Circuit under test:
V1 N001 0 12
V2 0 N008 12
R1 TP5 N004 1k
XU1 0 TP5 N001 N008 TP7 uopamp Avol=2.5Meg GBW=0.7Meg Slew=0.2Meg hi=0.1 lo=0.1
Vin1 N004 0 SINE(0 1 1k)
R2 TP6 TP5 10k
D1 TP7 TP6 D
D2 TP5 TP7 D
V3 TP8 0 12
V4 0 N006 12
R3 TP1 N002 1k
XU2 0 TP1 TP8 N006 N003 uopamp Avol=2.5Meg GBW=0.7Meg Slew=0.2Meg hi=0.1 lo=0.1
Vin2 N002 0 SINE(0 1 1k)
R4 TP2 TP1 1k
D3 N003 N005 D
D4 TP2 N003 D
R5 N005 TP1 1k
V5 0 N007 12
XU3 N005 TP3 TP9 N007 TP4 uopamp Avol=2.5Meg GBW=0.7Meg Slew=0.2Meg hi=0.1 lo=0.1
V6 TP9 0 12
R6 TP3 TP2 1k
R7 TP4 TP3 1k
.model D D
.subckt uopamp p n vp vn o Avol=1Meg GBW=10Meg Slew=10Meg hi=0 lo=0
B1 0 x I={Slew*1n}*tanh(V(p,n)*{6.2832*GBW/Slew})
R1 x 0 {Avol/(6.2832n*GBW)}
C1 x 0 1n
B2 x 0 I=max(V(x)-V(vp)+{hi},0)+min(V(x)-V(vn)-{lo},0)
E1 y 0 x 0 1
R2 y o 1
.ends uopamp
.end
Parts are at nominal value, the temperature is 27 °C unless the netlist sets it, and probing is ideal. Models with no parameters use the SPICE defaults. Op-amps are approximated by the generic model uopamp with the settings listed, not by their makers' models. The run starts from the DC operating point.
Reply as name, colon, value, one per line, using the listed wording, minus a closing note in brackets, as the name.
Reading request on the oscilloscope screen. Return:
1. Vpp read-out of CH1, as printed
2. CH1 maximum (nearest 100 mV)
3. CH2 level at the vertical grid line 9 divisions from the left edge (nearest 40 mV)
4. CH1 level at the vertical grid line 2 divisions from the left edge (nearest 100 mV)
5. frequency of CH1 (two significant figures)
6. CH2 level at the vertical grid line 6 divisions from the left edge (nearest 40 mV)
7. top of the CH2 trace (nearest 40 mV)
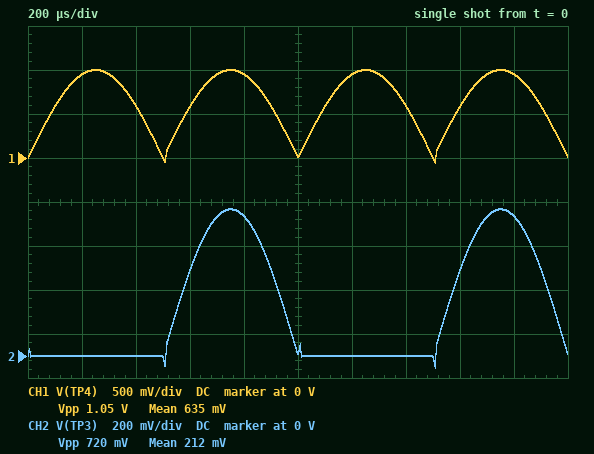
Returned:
Vpp read-out of CH1, as printed: 1.05 V
CH1 maximum: 1.0 V
CH2 level at the vertical grid line 9 divisions from the left edge: 640 mV
CH1 level at the vertical grid line 2 divisions from the left edge: 600 mV
frequency of CH1: 2.0 kHz
CH2 level at the vertical grid line 6 divisions from the left edge: 0 V
top of the CH2 trace: 680 mV
